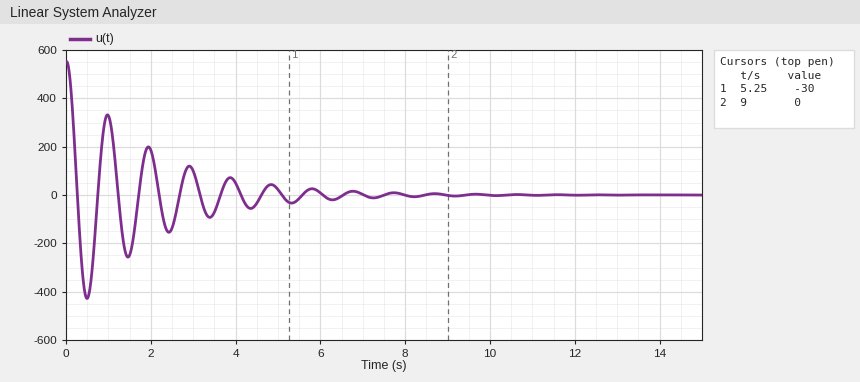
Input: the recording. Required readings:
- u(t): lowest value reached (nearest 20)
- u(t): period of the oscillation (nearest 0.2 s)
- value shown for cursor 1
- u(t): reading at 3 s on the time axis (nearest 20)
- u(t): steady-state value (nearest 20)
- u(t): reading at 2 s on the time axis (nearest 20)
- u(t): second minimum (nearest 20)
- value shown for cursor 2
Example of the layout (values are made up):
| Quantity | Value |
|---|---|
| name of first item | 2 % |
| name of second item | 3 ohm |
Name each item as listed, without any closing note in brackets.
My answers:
| Quantity | Value |
|---|---|
| u(t): lowest value reached | -420 |
| u(t): period of the oscillation | 1.0 s |
| value shown for cursor 1 | -30 |
| u(t): reading at 3 s on the time axis | 100 |
| u(t): steady-state value | 0 |
| u(t): reading at 2 s on the time axis | 180 |
| u(t): second minimum | -260 |
| value shown for cursor 2 | 0 |
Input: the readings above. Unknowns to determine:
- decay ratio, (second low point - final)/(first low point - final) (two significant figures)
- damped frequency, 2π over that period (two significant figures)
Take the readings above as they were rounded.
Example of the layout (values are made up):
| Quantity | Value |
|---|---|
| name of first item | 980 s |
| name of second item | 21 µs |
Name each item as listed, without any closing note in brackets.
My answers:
| Quantity | Value |
|---|---|
| decay ratio, (second low point - final)/(first low point - final) | 0.62 |
| damped frequency, 2π over that period | 6.3 rad/s |
